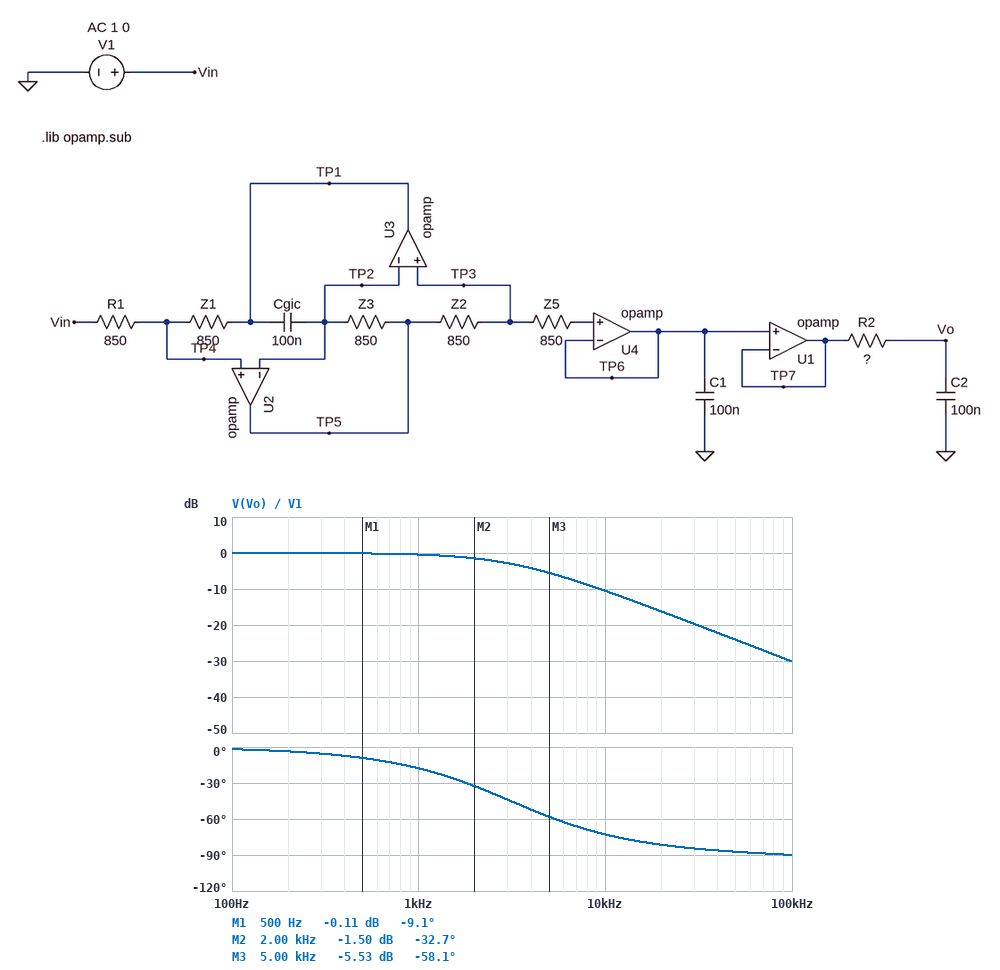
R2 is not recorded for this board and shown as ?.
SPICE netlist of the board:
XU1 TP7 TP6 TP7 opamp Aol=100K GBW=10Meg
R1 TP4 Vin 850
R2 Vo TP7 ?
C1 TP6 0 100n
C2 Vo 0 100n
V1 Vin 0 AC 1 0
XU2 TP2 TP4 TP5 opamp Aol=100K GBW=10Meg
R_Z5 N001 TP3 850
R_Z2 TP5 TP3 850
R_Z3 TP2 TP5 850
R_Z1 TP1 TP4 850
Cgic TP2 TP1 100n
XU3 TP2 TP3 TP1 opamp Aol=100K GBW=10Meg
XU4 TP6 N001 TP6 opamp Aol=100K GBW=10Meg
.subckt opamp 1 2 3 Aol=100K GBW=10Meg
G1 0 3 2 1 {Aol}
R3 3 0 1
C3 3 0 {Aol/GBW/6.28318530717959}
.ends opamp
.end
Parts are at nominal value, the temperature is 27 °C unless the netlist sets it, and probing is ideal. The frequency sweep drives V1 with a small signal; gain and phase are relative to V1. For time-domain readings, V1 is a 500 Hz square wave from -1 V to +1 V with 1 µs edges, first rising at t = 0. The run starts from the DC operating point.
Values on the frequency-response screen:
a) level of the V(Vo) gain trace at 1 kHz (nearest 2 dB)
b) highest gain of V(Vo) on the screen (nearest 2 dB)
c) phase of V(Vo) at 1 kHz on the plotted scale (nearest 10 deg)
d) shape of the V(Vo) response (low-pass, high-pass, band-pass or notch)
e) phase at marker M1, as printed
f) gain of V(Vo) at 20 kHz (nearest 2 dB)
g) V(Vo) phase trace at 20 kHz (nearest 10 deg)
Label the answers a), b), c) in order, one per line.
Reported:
a) 0 dB
b) 0 dB
c) -20 deg
d) low-pass
e) -9.1 deg
f) -16 dB
g) -80 deg
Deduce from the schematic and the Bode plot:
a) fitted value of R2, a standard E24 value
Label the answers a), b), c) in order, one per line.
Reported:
a) 510 Ω
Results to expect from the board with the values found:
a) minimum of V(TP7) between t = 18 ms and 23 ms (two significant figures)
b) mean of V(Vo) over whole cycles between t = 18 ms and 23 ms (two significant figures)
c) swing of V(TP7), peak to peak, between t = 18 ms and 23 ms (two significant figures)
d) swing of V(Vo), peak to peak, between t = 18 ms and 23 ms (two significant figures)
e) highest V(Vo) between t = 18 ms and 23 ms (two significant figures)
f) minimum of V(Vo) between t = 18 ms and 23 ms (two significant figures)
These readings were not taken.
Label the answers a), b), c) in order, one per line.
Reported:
a) -510 mV
b) 500 mV
c) 2.0 V
d) 2.0 V
e) 1.5 V
f) -500 mV
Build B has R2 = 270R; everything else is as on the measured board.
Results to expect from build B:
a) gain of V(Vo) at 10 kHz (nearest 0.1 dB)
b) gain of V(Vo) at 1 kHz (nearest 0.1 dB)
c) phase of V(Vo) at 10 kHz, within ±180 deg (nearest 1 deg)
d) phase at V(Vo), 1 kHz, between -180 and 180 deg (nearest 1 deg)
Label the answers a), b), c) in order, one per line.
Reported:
a) -5.9 dB
b) -0.1 dB
c) -60 deg
d) -10 deg
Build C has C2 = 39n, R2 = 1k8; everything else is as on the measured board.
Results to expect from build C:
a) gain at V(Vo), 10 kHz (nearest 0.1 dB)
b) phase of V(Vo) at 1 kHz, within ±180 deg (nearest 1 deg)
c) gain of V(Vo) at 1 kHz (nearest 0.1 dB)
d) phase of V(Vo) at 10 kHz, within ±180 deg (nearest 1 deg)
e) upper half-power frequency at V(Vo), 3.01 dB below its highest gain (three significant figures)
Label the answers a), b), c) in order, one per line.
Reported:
a) -13.1 dB
b) -24 deg
c) -0.8 dB
d) -77 deg
e) 2.27 kHz
